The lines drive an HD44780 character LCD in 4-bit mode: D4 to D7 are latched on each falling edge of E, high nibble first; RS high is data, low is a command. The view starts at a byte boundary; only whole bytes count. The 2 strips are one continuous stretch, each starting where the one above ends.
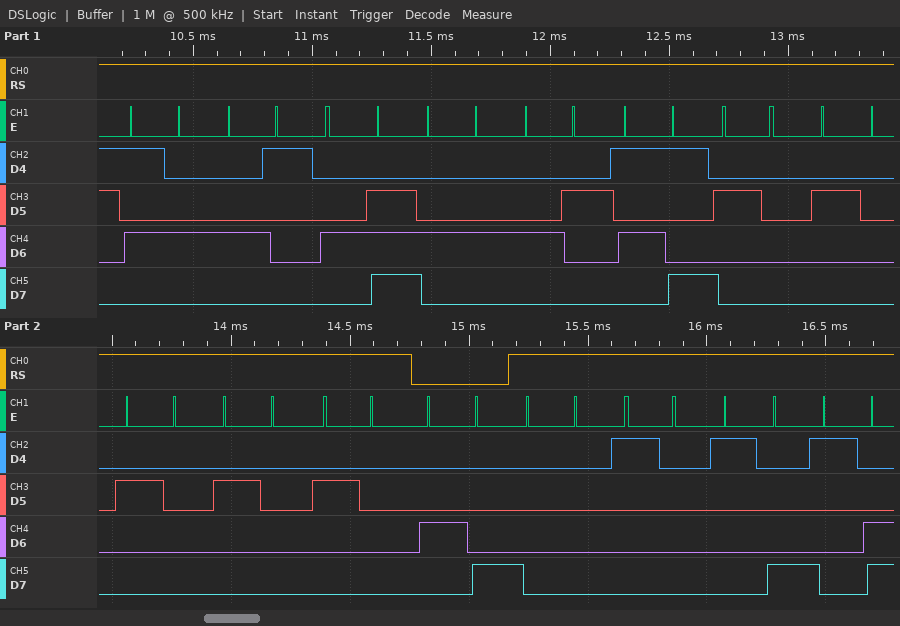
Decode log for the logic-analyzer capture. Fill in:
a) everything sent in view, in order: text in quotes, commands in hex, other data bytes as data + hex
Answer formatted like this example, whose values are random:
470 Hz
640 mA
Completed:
"TANDBY     " 0x48 data 00 10 18 1C
